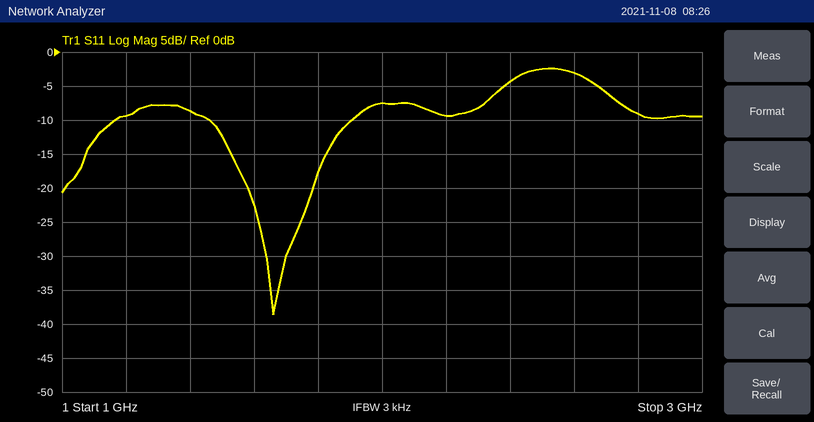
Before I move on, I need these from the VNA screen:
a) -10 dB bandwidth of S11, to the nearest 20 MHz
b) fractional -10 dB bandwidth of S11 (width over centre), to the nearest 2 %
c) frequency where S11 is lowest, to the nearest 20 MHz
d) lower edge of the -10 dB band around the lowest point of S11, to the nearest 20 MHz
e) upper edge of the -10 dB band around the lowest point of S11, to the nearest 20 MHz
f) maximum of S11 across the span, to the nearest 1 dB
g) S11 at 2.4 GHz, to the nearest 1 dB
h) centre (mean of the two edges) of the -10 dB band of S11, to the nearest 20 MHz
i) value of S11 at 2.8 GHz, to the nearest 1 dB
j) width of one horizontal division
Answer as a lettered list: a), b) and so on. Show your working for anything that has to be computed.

a) 1.90 GHz − 1.46 GHz = 440 MHz
b) 440 MHz / 1.68 GHz ≈ 26 %
c) 1.66 GHz
d) 1.46 GHz
e) 1.90 GHz
f) -2 dB
g) -4 dB
h) 1.68 GHz
i) -9 dB
j) 200 MHz
